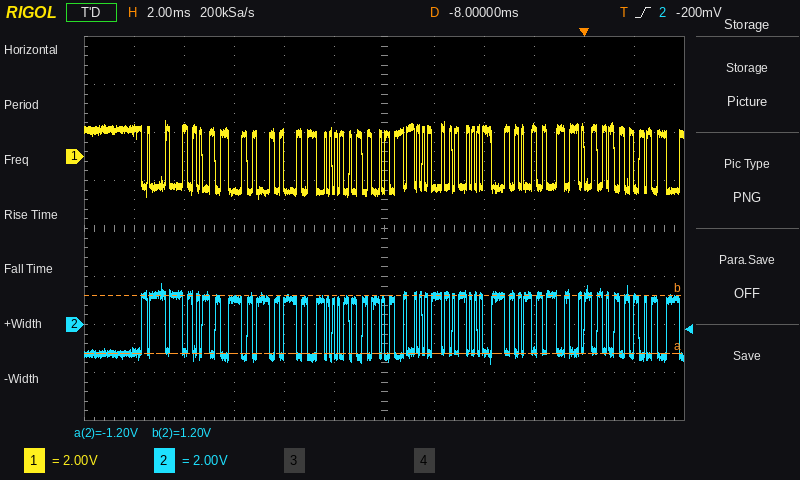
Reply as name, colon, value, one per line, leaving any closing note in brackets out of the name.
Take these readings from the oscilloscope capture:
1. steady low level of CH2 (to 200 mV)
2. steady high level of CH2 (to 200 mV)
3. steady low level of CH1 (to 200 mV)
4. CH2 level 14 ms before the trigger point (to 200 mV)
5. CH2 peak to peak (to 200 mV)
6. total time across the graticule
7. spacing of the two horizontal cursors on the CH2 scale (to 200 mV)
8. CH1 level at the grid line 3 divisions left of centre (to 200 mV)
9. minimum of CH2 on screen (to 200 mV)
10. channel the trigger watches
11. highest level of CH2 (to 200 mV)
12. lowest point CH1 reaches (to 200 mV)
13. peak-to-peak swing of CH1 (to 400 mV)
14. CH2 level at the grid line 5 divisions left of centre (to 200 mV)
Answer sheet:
steady low level of CH2: -1.2 V
steady high level of CH2: 1.2 V
steady low level of CH1: -1.4 V
CH2 level 14 ms before the trigger point: 1.0 V
CH2 peak to peak: 3.4 V
total time across the graticule: 24 ms
spacing of the two horizontal cursors on the CH2 scale: 2.4 V
CH1 level at the grid line 3 divisions left of centre: -1.4 V
minimum of CH2 on screen: -1.6 V
channel the trigger watches: CH2
highest level of CH2: 1.8 V
lowest point CH1 reaches: -1.8 V
peak-to-peak swing of CH1: 3.2 V
CH2 level at the grid line 5 divisions left of centre: -1.2 V
